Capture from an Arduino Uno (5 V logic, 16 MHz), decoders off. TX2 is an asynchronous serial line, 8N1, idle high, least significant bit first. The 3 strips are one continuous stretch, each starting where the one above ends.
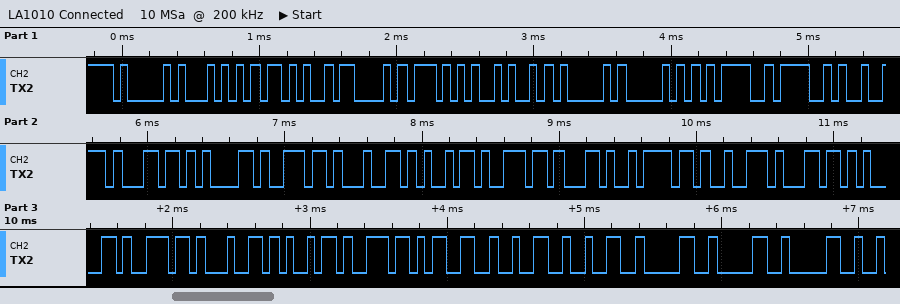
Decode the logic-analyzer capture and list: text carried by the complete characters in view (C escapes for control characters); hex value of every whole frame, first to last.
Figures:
"AT+CWJAP=Orlandin,orlandin322000"
41 54 2B 43 57 4A 41 50 3D 4F 72 6C 61 6E 64 69 6E 2C 6F 72 6C 61 6E 64 69 6E 33 32 32 30 30 30
